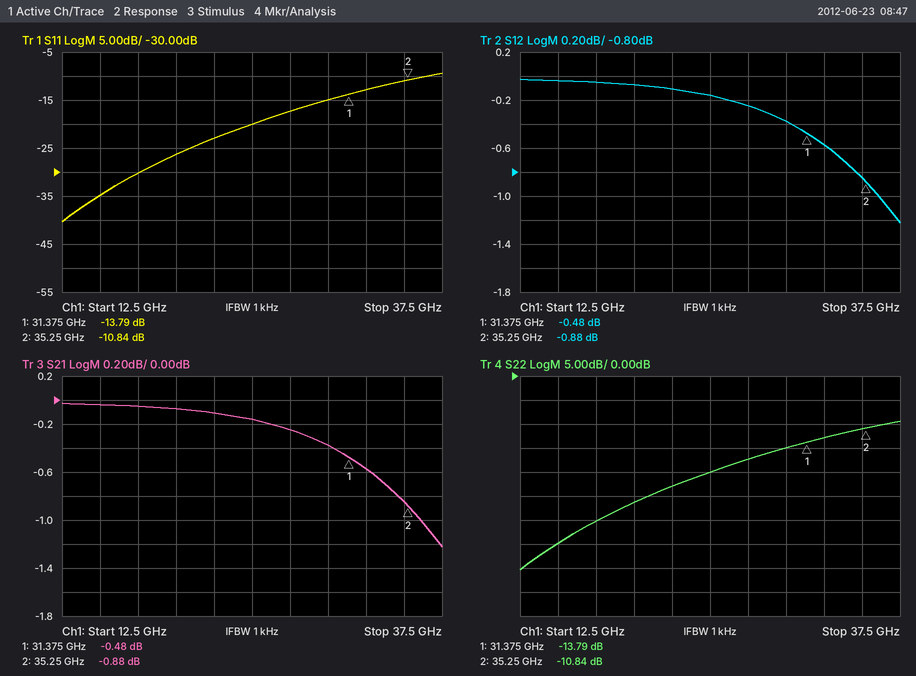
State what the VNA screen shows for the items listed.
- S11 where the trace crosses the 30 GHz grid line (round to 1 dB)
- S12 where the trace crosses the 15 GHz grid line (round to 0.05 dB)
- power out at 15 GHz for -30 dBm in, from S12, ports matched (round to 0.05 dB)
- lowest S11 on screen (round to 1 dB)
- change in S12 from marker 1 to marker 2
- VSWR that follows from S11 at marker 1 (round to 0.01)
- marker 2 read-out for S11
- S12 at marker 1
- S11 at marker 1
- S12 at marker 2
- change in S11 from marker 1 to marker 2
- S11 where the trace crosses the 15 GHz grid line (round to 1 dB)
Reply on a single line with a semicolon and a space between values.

-15 dB; -0.05 dB; -30.05 dBm; -40 dB; -0.40 dB; 1.51; -10.84 dB; -0.48 dB; -13.79 dB; -0.88 dB; 2.95 dB; -35 dB
